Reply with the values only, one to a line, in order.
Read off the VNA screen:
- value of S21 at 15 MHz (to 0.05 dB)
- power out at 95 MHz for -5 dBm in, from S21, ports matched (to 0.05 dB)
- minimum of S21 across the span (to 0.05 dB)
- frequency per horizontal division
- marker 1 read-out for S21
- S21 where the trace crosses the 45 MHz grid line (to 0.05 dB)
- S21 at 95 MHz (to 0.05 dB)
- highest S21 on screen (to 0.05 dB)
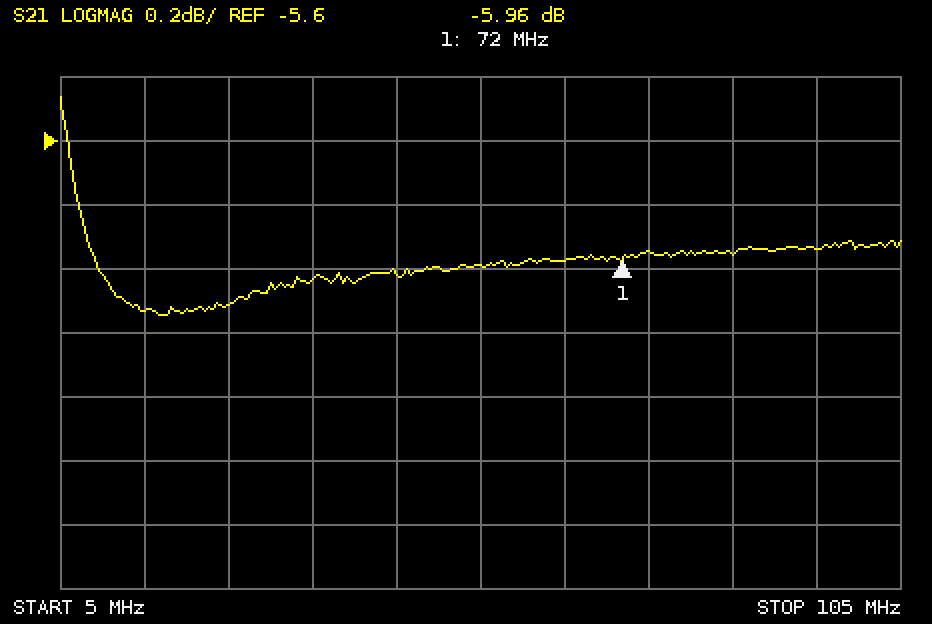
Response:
-6.15 dB
-10.95 dBm
-6.15 dB
10 MHz
-5.96 dB
-6.00 dB
-5.95 dB
-5.45 dB
